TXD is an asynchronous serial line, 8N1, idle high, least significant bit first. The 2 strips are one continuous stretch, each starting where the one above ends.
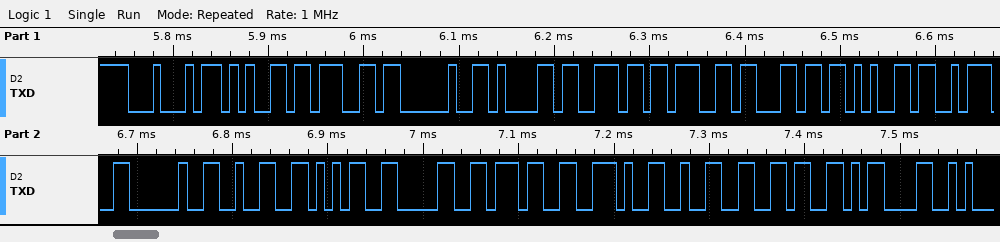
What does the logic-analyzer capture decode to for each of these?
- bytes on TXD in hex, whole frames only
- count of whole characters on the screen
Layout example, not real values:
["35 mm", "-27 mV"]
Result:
["44 65 67 20 61 6E 67 6C 65 3A 20 32 35 30 37 2E 32 36 0D", "19"]
